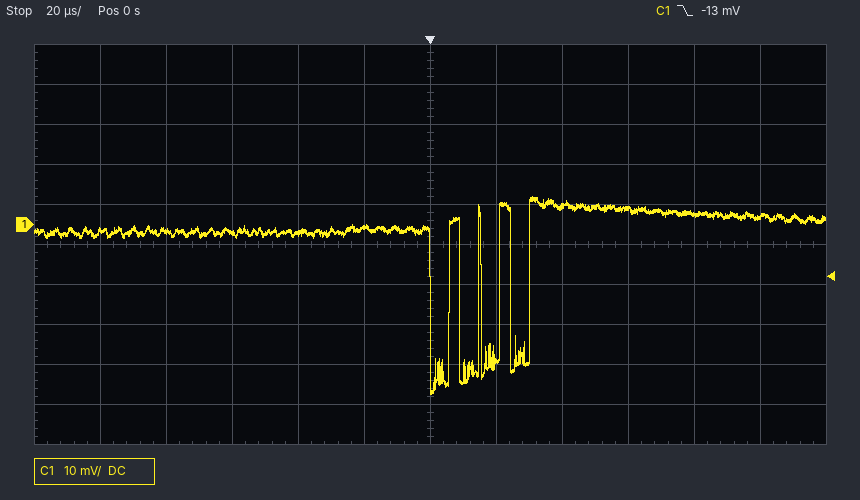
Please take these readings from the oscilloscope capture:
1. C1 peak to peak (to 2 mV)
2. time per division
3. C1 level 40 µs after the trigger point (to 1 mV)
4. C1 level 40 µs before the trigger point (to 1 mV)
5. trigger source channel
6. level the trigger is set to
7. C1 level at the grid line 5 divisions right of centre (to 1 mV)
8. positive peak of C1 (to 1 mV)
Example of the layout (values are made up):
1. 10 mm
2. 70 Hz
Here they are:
1. 50 mV
2. 20 µs
3. 4 mV
4. -2 mV
5. C1
6. -13 mV
7. 2 mV
8. 7 mV
